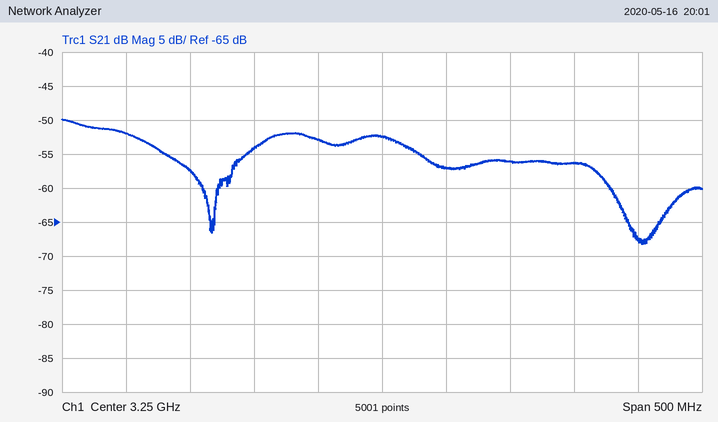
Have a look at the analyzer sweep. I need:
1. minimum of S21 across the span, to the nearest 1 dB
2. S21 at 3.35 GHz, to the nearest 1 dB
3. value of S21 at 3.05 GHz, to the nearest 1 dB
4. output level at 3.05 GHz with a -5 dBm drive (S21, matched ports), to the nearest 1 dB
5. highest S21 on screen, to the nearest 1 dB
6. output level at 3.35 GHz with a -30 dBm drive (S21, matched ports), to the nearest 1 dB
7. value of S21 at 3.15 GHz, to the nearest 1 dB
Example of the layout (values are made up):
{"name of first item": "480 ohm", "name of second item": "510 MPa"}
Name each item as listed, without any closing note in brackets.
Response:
{"minimum of S21 across the span, to the nearest 1 dB": "-68 dB", "S21 at 3.35 GHz, to the nearest 1 dB": "-56 dB", "value of S21 at 3.05 GHz, to the nearest 1 dB": "-52 dB", "output level at 3.05 GHz with a -5 dBm drive (S21, matched ports), to the nearest 1 dB": "-57 dBm", "highest S21 on screen, to the nearest 1 dB": "-50 dB", "output level at 3.35 GHz with a -30 dBm drive (S21, matched ports), to the nearest 1 dB": "-86 dBm", "value of S21 at 3.15 GHz, to the nearest 1 dB": "-54 dB"}
